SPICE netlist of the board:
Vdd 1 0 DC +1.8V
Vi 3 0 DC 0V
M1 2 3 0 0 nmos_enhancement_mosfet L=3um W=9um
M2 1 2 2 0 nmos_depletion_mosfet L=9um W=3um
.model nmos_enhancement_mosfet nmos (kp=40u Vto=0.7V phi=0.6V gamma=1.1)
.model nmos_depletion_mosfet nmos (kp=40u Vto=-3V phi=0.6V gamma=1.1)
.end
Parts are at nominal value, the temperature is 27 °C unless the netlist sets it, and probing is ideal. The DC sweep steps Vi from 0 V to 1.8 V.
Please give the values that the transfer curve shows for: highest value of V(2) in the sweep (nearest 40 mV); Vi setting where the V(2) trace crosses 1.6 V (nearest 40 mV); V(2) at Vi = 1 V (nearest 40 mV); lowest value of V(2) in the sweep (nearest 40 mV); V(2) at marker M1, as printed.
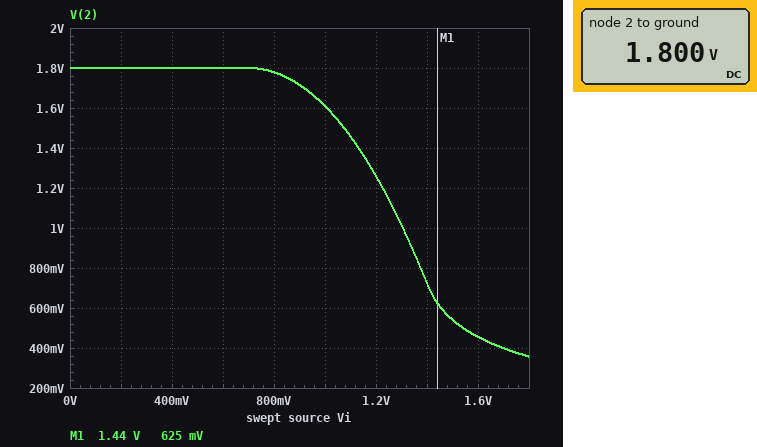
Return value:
1.80 V
1.00 V
1.60 V
360 mV
625 mV
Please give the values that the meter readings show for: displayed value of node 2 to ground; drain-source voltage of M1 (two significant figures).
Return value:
1.800 V
1.8 V
